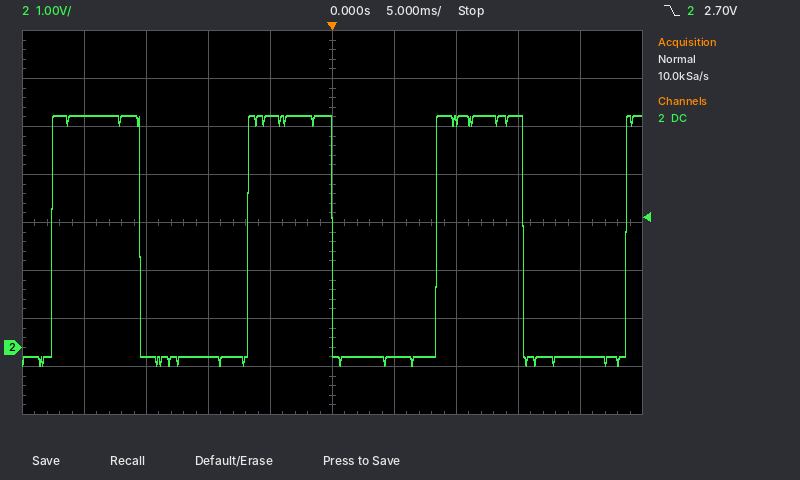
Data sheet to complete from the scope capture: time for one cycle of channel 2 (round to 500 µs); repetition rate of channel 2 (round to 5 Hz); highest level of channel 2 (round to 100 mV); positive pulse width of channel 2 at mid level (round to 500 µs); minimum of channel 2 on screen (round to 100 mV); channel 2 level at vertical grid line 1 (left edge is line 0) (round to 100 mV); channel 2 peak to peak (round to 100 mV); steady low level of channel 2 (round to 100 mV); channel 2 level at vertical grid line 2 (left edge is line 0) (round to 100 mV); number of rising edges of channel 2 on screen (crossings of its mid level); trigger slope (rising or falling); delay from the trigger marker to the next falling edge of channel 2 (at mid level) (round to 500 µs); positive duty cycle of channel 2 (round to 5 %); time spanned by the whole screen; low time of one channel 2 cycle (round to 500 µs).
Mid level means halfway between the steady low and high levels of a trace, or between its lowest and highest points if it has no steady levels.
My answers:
15.5 ms
65 Hz
4.8 V
7.0 ms
-400 mV
4.8 V
5.2 V
-200 mV
-200 mV
4
falling
15.5 ms
45 %
50 ms
8.5 ms
